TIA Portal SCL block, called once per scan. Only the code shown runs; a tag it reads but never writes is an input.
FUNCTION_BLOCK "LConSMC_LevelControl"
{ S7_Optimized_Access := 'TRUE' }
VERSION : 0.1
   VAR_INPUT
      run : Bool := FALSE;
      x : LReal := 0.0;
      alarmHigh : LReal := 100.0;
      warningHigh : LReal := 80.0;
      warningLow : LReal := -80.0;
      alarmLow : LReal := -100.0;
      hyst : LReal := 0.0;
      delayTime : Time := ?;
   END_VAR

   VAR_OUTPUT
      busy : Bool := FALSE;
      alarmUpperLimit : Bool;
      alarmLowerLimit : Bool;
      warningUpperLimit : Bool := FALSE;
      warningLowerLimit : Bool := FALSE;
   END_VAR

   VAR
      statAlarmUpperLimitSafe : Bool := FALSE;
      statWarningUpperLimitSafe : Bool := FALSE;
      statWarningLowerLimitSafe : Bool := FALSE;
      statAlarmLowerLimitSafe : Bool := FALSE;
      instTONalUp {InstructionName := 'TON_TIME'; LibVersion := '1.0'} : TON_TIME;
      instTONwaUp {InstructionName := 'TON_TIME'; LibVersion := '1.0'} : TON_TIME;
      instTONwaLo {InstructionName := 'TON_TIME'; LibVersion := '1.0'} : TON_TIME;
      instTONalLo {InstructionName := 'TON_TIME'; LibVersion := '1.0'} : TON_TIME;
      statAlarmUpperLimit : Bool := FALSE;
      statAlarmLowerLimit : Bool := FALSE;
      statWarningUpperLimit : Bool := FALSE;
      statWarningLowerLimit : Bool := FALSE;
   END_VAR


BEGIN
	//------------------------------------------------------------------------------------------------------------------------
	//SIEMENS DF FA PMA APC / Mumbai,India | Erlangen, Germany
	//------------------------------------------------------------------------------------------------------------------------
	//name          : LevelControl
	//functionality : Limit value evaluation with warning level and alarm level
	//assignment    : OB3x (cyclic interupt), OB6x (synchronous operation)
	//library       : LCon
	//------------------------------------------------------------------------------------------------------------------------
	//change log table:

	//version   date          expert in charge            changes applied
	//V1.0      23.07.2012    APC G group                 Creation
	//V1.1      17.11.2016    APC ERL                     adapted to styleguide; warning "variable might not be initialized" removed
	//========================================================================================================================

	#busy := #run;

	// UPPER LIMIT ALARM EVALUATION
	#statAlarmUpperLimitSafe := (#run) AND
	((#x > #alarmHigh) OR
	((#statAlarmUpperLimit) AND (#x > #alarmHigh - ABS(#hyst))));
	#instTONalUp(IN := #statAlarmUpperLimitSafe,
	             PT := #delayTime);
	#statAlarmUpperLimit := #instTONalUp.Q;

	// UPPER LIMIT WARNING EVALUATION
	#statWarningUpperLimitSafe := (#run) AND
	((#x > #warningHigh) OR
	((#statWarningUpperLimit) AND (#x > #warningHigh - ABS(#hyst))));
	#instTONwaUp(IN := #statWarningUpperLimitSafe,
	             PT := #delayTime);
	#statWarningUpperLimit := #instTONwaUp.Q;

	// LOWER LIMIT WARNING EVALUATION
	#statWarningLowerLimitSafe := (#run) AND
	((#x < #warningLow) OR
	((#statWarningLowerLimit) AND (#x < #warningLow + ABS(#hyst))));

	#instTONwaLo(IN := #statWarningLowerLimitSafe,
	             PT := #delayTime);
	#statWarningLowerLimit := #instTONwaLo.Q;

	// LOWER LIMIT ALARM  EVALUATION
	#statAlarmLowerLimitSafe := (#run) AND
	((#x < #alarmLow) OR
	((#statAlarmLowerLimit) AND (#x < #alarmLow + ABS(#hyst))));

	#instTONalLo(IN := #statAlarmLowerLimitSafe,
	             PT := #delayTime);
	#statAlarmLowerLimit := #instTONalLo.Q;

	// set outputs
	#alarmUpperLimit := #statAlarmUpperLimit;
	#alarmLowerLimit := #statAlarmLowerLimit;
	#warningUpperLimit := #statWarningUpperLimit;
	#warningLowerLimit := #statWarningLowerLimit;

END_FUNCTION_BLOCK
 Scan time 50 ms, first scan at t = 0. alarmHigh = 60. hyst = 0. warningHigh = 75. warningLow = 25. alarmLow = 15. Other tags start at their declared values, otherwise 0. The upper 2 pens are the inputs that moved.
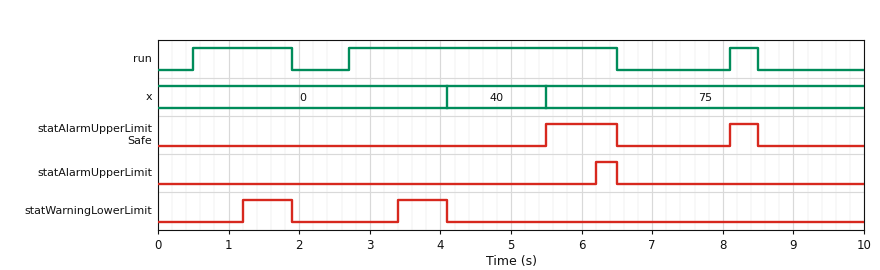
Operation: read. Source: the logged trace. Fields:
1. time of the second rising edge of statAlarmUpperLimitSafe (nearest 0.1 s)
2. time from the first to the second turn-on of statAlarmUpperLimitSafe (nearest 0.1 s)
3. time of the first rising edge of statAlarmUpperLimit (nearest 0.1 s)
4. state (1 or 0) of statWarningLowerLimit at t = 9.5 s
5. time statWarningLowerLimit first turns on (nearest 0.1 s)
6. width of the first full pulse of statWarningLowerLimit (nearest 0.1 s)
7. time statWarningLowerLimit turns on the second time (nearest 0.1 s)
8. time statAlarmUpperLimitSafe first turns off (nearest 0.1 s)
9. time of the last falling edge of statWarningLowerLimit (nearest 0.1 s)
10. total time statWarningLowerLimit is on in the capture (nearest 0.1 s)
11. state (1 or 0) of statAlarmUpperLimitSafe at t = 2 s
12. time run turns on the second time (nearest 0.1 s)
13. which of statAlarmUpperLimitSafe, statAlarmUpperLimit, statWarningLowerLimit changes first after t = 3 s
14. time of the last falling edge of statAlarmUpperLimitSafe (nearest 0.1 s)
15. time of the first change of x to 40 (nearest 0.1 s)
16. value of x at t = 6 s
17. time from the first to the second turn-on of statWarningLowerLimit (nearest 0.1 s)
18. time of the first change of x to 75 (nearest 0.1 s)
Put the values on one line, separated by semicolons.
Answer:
8.1 s; 2.6 s; 6.2 s; 0; 1.2 s; 0.7 s; 3.4 s; 6.5 s; 4.1 s; 1.4 s; 0; 2.7 s; statWarningLowerLimit; 8.5 s; 4.1 s; 75; 2.2 s; 5.5 s
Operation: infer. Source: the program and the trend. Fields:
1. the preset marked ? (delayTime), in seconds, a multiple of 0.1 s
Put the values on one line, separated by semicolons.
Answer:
0.7 s
